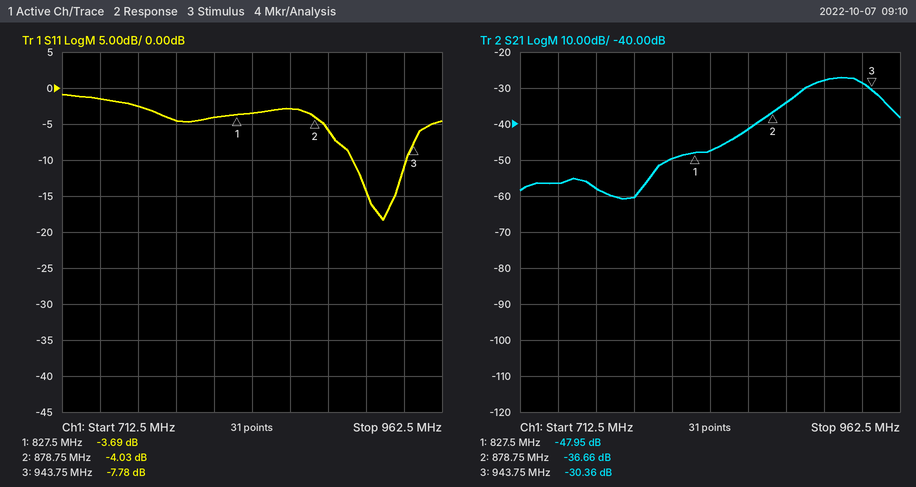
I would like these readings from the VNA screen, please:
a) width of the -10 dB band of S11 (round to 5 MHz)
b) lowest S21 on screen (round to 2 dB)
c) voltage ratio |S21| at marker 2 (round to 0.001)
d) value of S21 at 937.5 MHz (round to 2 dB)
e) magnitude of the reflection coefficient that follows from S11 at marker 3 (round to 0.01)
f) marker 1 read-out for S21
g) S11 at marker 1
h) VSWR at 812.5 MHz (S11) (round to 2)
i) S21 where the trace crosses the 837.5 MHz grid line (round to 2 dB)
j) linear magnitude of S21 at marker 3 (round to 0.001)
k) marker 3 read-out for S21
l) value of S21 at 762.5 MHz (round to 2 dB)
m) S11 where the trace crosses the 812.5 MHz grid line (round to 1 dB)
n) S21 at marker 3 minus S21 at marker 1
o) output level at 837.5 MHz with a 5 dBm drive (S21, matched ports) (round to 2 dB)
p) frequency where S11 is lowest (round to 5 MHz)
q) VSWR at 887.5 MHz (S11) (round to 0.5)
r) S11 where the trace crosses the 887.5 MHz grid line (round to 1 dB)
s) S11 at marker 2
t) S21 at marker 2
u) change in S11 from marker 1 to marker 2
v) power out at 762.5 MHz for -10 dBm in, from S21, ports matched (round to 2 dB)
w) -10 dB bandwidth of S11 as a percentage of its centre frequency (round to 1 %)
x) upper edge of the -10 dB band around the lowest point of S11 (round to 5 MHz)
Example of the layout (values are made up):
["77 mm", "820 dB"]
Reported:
["35 MHz", "-60 dB", "0.015", "-28 dB", "0.41", "-47.95 dB", "-3.69 dB", "4", "-48 dB", "0.030", "-30.36 dB", "-58 dB", "-4 dB", "17.59 dB", "-42 dBm", "925 MHz", "3.0", "-6 dB", "-4.03 dB", "-36.66 dB", "-0.34 dB", "-68 dBm", "4 %", "940 MHz"]
